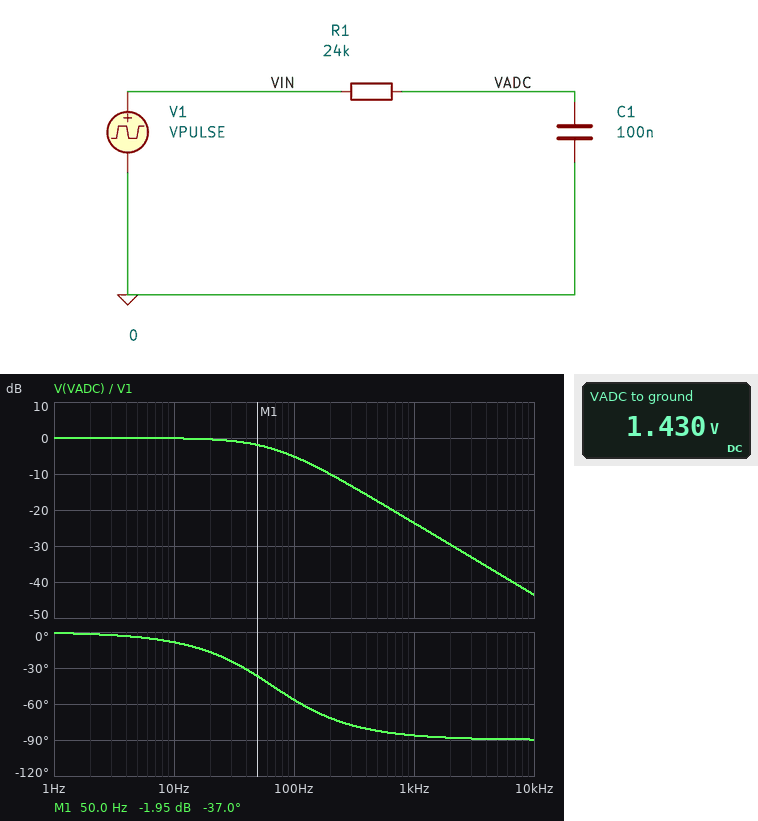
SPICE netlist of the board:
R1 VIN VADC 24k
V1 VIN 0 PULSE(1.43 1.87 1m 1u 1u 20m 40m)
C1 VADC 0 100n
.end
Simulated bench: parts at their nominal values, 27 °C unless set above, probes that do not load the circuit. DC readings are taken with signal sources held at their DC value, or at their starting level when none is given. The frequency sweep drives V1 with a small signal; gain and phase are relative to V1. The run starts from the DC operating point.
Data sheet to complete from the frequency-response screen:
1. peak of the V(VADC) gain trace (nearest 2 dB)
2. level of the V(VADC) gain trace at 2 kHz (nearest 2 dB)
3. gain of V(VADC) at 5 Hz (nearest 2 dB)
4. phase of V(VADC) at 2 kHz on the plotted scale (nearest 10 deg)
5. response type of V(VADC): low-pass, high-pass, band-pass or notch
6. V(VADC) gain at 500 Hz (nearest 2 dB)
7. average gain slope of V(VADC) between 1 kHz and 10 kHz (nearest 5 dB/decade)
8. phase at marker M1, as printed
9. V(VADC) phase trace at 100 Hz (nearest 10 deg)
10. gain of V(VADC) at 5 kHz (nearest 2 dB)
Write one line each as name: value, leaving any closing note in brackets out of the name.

peak of the V(VADC) gain trace: 0 dB
level of the V(VADC) gain trace at 2 kHz: -30 dB
gain of V(VADC) at 5 Hz: 0 dB
phase of V(VADC) at 2 kHz on the plotted scale: -90 deg
response type of V(VADC): low-pass, high-pass, band-pass or notch: low-pass
V(VADC) gain at 500 Hz: -18 dB
average gain slope of V(VADC) between 1 kHz and 10 kHz: -20 dB/decade
phase at marker M1, as printed: -37.0 deg
V(VADC) phase trace at 100 Hz: -60 deg
gain of V(VADC) at 5 kHz: -38 dB
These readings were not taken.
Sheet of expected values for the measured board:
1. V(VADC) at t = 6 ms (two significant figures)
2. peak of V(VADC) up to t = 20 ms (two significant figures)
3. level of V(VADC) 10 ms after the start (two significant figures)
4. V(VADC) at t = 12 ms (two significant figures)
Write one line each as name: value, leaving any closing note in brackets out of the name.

V(VADC) at t = 6 ms: 1.8 V
peak of V(VADC) up to t = 20 ms: 1.9 V
level of V(VADC) 10 ms after the start: 1.9 V
V(VADC) at t = 12 ms: 1.9 V
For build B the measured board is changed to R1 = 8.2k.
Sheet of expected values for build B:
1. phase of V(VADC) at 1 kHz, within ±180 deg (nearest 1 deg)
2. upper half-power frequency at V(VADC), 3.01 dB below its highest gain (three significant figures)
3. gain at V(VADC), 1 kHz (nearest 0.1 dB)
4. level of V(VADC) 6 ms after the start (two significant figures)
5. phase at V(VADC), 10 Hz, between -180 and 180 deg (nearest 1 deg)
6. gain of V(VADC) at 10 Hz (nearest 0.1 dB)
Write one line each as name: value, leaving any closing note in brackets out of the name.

phase of V(VADC) at 1 kHz, within ±180 deg: -79 deg
upper half-power frequency at V(VADC), 3.01 dB below its highest gain: 194 Hz
gain at V(VADC), 1 kHz: -14.4 dB
level of V(VADC) 6 ms after the start: 1.9 V
phase at V(VADC), 10 Hz, between -180 and 180 deg: -3 deg
gain of V(VADC) at 10 Hz: 0 dB
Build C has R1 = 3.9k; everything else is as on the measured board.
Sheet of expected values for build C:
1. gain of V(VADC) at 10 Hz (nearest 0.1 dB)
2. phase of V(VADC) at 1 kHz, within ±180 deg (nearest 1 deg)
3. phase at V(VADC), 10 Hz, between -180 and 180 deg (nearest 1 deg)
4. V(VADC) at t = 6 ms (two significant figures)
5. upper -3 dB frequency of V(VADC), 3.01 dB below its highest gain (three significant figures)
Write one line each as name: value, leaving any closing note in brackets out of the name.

gain of V(VADC) at 10 Hz: 0 dB
phase of V(VADC) at 1 kHz, within ±180 deg: -68 deg
phase at V(VADC), 10 Hz, between -180 and 180 deg: -1 deg
V(VADC) at t = 6 ms: 1.9 V
upper -3 dB frequency of V(VADC), 3.01 dB below its highest gain: 408 Hz
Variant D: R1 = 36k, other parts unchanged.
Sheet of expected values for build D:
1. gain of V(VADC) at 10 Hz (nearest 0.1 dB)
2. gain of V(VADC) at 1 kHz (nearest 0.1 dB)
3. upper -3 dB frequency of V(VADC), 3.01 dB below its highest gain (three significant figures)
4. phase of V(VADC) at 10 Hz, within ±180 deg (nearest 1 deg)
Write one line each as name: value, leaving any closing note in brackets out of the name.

gain of V(VADC) at 10 Hz: -0.2 dB
gain of V(VADC) at 1 kHz: -27.1 dB
upper -3 dB frequency of V(VADC), 3.01 dB below its highest gain: 44.2 Hz
phase of V(VADC) at 10 Hz, within ±180 deg: -13 deg
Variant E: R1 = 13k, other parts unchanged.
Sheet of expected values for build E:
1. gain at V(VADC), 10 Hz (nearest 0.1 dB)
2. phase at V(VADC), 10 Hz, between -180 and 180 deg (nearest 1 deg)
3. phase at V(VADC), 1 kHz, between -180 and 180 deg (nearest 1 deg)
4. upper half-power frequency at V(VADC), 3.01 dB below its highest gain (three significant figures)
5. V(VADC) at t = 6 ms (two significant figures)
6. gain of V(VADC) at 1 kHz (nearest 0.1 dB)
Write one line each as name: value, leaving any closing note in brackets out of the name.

gain at V(VADC), 10 Hz: 0 dB
phase at V(VADC), 10 Hz, between -180 and 180 deg: -5 deg
phase at V(VADC), 1 kHz, between -180 and 180 deg: -83 deg
upper half-power frequency at V(VADC), 3.01 dB below its highest gain: 122 Hz
V(VADC) at t = 6 ms: 1.9 V
gain of V(VADC) at 1 kHz: -18.3 dB
